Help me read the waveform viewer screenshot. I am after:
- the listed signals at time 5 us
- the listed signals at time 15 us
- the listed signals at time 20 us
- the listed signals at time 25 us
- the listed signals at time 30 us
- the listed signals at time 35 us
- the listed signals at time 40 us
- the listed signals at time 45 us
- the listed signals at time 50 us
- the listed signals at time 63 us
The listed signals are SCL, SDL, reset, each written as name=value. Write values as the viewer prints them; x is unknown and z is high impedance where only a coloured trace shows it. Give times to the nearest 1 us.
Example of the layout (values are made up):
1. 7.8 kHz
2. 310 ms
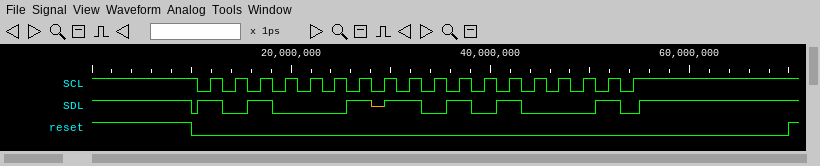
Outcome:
1. SCL=1, SDL=1, reset=1
2. SCL=1, SDL=0, reset=0
3. SCL=1, SDL=0, reset=0
4. SCL=1, SDL=0, reset=0
5. SCL=1, SDL=1, reset=0
6. SCL=1, SDL=0, reset=0
7. SCL=1, SDL=0, reset=0
8. SCL=1, SDL=0, reset=0
9. SCL=1, SDL=0, reset=0
10. SCL=1, SDL=1, reset=0
